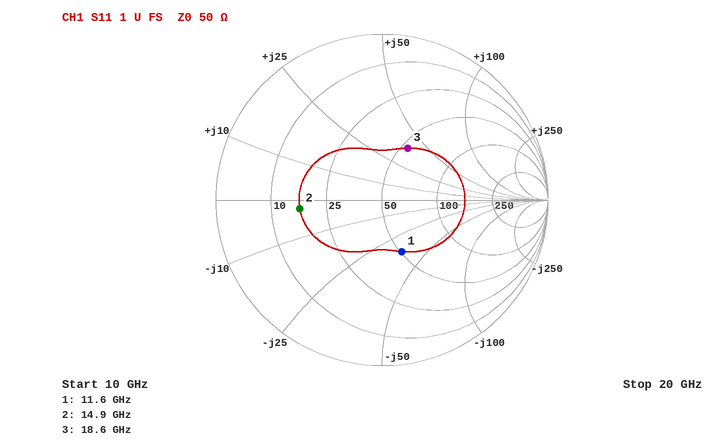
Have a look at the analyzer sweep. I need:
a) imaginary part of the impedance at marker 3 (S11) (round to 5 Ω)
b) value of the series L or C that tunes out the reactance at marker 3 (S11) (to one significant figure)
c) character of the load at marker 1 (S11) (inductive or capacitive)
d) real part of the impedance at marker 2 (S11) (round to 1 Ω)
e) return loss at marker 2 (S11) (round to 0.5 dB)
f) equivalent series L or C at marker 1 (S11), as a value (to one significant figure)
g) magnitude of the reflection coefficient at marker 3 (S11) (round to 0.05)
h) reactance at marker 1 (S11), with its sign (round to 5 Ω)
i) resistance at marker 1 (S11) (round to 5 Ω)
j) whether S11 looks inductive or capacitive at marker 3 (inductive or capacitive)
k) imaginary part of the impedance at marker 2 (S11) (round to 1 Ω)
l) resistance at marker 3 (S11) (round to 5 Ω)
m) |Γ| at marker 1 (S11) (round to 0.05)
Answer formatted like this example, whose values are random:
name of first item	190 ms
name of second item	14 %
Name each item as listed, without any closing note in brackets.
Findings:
imaginary part of the impedance at marker 3 (S11)	+40 Ω
value of the series L or C that tunes out the reactance at marker 3 (S11)	200 fF
character of the load at marker 1 (S11)	capacitive
real part of the impedance at marker 2 (S11)	17 Ω
return loss at marker 2 (S11)	6.0 dB
equivalent series L or C at marker 1 (S11), as a value	400 fF
magnitude of the reflection coefficient at marker 3 (S11)	0.35
reactance at marker 1 (S11), with its sign	-35 Ω
resistance at marker 1 (S11)	50 Ω
whether S11 looks inductive or capacitive at marker 3	inductive
imaginary part of the impedance at marker 2 (S11)	-2 Ω
resistance at marker 3 (S11)	55 Ω
|Γ| at marker 1 (S11)	0.35
